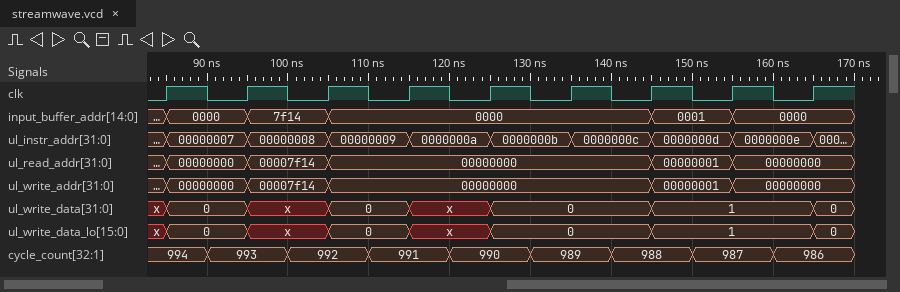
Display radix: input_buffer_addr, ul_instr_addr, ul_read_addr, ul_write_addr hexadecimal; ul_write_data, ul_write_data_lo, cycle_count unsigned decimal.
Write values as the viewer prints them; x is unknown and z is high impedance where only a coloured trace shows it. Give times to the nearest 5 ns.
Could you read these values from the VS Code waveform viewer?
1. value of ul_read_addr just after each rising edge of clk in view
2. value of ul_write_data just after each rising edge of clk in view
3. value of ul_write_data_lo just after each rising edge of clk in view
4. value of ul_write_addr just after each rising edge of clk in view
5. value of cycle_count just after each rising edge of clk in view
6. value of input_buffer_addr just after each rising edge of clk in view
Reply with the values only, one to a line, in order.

00000000, 00007f14, 00000000, 00000000, 00000000, 00000000, 00000001, 00000000, 00000000
0, x, 0, x, 0, 0, 1, 1, 0
0, x, 0, x, 0, 0, 1, 1, 0
00000000, 00007f14, 00000000, 00000000, 00000000, 00000000, 00000001, 00000000, 00000000
994, 993, 992, 991, 990, 989, 988, 987, 986
0000, 7f14, 0000, 0000, 0000, 0000, 0001, 0000, 0000
